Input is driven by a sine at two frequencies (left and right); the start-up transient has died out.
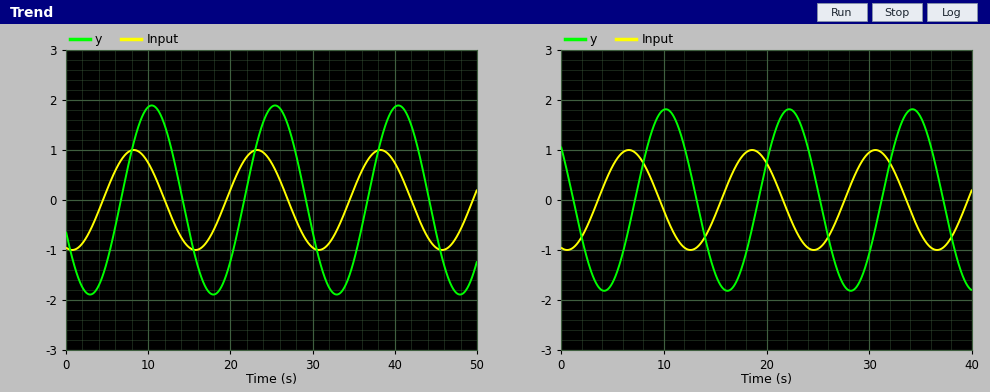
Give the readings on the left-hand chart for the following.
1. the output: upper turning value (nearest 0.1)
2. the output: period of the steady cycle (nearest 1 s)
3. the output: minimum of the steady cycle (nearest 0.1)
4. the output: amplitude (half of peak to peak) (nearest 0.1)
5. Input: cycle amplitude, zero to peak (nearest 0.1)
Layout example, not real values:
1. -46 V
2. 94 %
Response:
1. 1.9
2. 15 s
3. -1.9
4. 1.9
5. 1.0
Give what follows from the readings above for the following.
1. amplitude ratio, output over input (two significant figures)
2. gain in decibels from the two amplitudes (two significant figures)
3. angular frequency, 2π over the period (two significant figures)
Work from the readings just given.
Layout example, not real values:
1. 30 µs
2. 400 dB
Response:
1. 1.9
2. 5.6 dB
3. 0.42 rad/s
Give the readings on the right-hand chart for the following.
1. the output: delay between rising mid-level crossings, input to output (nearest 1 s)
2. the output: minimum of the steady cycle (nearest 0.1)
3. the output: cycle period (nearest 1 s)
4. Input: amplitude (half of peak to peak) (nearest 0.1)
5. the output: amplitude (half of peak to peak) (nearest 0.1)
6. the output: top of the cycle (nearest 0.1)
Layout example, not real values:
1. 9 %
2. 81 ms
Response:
1. 4 s
2. -1.8
3. 12 s
4. 1.0
5. 1.8
6. 1.8
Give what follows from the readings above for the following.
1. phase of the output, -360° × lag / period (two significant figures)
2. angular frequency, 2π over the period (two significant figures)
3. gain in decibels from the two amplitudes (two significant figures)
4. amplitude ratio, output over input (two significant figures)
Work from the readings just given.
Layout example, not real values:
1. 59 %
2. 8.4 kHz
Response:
1. -120°
2. 0.52 rad/s
3. 5.1 dB
4. 1.8
